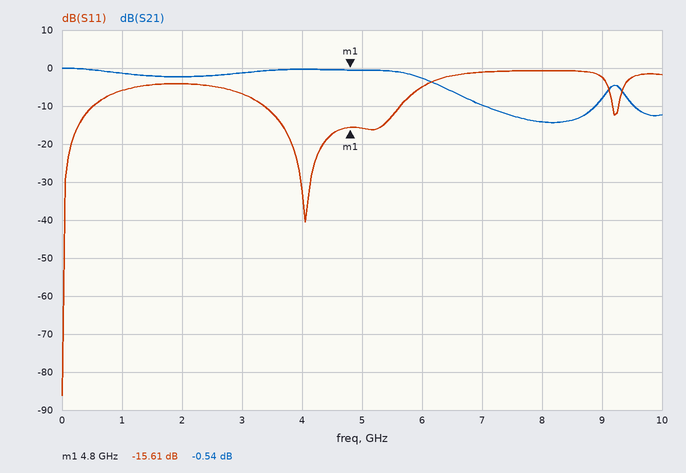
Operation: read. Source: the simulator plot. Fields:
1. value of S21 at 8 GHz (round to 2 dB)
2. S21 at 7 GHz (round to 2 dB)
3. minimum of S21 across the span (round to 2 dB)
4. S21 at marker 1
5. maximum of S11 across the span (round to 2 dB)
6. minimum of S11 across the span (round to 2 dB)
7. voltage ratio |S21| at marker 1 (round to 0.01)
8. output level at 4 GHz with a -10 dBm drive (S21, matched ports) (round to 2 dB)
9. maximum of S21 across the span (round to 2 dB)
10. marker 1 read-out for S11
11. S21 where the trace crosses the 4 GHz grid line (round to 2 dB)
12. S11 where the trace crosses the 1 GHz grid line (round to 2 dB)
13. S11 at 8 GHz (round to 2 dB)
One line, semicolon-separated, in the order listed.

-14 dB; -10 dB; -14 dB; -0.54 dB; 0 dB; -86 dB; 0.94; -10 dBm; 0 dB; -15.61 dB; 0 dB; -6 dB; 0 dB
